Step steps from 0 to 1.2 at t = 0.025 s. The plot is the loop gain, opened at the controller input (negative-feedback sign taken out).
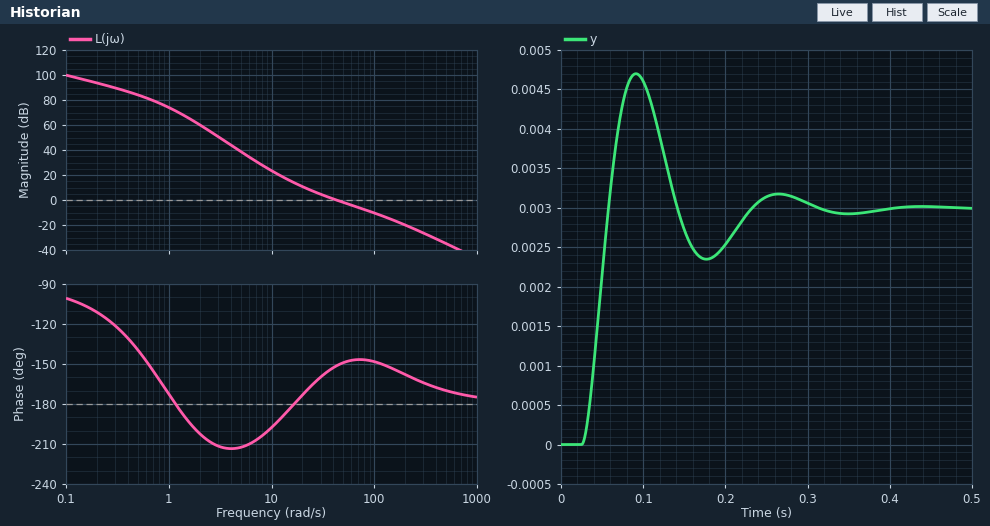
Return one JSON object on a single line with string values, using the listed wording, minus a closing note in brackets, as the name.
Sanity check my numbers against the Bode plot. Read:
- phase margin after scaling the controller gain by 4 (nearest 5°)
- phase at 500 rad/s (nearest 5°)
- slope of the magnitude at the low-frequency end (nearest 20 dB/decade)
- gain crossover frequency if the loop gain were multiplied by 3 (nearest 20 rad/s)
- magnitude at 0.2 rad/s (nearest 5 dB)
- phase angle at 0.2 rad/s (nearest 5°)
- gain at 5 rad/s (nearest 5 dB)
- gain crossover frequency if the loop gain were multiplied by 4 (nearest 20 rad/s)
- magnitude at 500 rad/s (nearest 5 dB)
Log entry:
{"phase margin after scaling the controller gain by 4": "30°", "phase at 500 rad/s": "-170°", "slope of the magnitude at the low-frequency end": "-20 dB/decade", "gain crossover frequency if the loop gain were multiplied by 3": "100 rad/s", "magnitude at 0.2 rad/s": "95 dB", "phase angle at 0.2 rad/s": "-110°", "gain at 5 rad/s": "40 dB", "gain crossover frequency if the loop gain were multiplied by 4": "120 rad/s", "magnitude at 500 rad/s": "-35 dB"}
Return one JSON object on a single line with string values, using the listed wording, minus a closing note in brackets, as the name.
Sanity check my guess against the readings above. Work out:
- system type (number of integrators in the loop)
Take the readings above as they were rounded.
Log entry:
{"system type": "1"}
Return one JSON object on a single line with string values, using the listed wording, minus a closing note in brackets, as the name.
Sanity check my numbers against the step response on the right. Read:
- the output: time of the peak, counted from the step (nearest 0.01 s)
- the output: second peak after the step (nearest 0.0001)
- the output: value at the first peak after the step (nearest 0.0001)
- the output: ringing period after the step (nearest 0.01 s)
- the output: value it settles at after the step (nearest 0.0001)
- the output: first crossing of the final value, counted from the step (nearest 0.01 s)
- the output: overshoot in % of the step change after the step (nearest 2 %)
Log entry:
{"the output: time of the peak, counted from the step": "0.07 s", "the output: second peak after the step": "0.0032", "the output: value at the first peak after the step": "0.0047", "the output: ringing period after the step": "0.17 s", "the output: value it settles at after the step": "0.0030", "the output: first crossing of the final value, counted from the step": "0.03 s", "the output: overshoot in % of the step change after the step": "56 %"}
